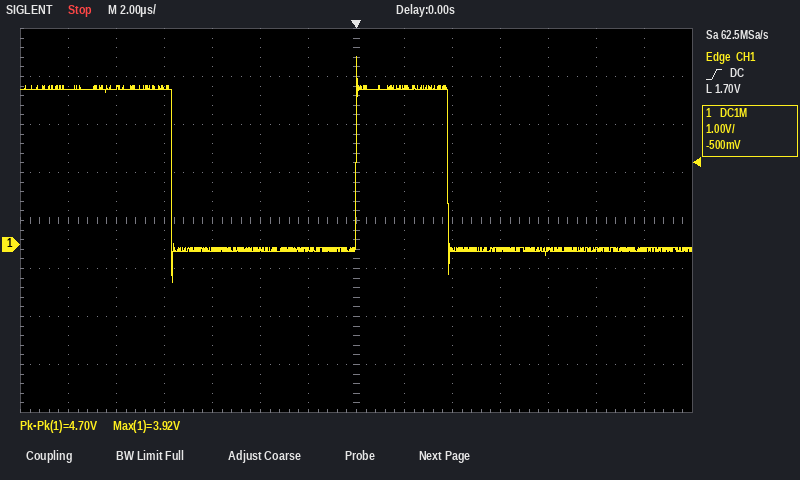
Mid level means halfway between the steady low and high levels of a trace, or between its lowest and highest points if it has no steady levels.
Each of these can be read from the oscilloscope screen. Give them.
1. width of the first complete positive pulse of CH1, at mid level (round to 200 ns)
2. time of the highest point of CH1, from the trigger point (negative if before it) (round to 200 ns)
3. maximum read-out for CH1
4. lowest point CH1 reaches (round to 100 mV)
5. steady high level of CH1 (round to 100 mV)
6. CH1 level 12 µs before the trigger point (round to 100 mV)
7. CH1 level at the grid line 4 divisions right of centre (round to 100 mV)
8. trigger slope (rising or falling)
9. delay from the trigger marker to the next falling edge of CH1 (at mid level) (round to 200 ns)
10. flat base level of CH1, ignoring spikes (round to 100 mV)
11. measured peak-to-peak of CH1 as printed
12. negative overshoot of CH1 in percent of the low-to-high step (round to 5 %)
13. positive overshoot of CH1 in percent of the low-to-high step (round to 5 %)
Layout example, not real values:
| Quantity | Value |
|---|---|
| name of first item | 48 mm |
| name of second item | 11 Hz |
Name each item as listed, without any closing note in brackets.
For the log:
| Quantity | Value |
|---|---|
| width of the first complete positive pulse of CH1, at mid level | 3.8 µs |
| time of the highest point of CH1, from the trigger point (negative if before it) | 0.0 µs |
| maximum read-out for CH1 | 3.92 V |
| lowest point CH1 reaches | -800 mV |
| steady high level of CH1 | 3.2 V |
| CH1 level 12 µs before the trigger point | 3.2 V |
| CH1 level at the grid line 4 divisions right of centre | -100 mV |
| trigger slope | rising |
| delay from the trigger marker to the next falling edge of CH1 (at mid level) | 3.8 µs |
| flat base level of CH1, ignoring spikes | -100 mV |
| measured peak-to-peak of CH1 as printed | 4.70 V |
| negative overshoot of CH1 in percent of the low-to-high step | 20 % |
| positive overshoot of CH1 in percent of the low-to-high step | 20 % |
